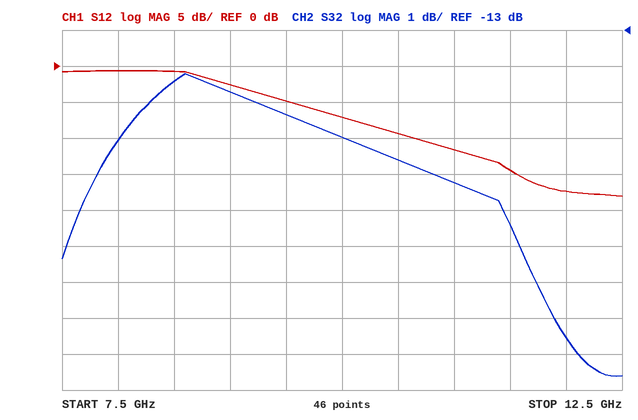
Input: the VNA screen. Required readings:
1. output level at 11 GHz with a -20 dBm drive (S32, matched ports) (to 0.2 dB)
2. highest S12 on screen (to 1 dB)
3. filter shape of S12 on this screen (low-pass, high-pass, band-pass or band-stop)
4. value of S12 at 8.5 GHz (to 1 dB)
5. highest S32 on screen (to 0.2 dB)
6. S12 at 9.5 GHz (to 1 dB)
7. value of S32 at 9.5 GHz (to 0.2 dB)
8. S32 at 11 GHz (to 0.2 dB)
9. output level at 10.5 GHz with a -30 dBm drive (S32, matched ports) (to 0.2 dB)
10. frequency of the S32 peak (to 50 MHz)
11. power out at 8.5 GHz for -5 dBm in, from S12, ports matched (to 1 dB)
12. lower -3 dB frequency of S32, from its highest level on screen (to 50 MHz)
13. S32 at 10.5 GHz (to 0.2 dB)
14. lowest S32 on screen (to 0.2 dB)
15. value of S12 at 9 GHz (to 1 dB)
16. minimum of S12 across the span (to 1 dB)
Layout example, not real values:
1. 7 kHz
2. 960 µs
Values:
1. -37.2 dBm
2. -1 dB
3. low-pass
4. -1 dB
5. -14.2 dB
6. -5 dB
7. -15.4 dB
8. -17.2 dB
9. -46.6 dBm
10. 8.60 GHz
11. -6 dBm
12. 7.80 GHz
13. -16.6 dB
14. -22.6 dB
15. -3 dB
16. -18 dB
